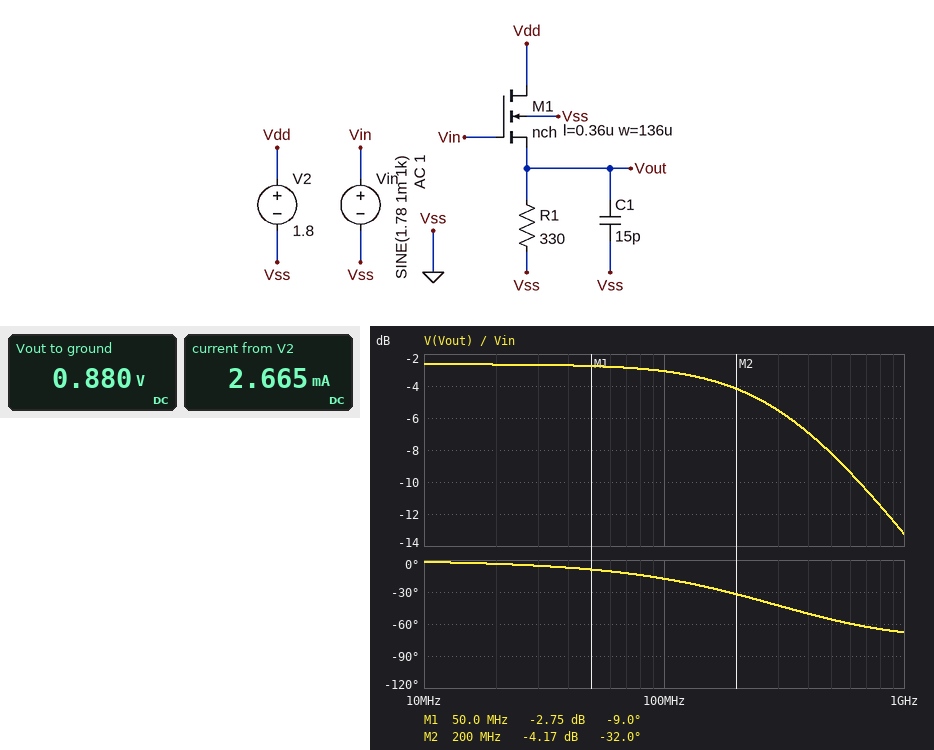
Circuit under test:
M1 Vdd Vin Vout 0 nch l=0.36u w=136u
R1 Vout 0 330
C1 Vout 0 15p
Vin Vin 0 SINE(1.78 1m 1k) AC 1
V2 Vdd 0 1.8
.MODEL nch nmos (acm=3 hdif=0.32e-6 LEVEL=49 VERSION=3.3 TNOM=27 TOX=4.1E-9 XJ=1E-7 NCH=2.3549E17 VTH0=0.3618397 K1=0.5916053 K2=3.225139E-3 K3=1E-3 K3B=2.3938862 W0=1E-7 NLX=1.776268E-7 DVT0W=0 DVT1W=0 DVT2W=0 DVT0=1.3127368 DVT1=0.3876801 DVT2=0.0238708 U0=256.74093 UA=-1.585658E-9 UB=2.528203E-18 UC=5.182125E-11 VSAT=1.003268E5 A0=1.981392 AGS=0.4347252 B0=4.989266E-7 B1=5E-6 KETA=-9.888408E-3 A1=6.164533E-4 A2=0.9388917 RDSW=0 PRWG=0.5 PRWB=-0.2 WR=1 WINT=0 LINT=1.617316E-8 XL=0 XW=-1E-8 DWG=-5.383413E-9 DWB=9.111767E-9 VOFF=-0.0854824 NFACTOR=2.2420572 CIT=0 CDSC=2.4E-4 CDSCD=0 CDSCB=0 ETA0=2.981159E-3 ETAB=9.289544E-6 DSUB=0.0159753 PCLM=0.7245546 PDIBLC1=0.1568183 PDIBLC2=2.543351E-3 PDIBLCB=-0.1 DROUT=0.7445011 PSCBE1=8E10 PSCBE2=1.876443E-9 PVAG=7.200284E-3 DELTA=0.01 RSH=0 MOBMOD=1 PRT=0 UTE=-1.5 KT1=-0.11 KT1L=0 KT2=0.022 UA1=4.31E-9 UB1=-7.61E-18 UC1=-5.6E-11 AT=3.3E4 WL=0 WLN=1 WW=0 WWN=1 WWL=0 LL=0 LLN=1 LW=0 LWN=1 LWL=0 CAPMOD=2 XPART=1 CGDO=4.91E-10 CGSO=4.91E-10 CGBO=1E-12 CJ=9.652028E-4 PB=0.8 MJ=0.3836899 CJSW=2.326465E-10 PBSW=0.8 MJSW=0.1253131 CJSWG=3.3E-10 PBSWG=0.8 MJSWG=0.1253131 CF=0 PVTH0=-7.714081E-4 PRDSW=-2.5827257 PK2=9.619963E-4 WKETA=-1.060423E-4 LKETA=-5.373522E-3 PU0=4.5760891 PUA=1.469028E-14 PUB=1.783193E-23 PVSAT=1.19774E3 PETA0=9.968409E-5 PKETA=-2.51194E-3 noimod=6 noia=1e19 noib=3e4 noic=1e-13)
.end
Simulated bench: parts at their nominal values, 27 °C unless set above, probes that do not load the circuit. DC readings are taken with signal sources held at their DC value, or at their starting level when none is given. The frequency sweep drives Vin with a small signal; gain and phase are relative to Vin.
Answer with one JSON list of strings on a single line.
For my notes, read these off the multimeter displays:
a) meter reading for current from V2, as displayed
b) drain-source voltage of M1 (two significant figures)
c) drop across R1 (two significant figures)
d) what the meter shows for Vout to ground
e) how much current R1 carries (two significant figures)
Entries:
["2.665 mA", "920 mV", "880 mV", "0.880 V", "2.7 mA"]
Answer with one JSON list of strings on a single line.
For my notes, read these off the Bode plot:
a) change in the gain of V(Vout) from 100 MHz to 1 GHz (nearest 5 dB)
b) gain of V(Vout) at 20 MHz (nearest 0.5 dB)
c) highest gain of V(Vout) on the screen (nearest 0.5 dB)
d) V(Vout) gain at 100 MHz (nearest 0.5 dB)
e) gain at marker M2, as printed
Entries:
["-10 dB", "-2.5 dB", "-2.5 dB", "-3.0 dB", "-4.17 dB"]
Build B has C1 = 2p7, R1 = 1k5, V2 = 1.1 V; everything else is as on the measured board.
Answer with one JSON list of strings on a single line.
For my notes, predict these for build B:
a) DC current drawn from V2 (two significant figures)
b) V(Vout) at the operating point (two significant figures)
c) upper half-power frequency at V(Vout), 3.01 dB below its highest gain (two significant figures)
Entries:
["650 µA", "970 mV", "670 MHz"]
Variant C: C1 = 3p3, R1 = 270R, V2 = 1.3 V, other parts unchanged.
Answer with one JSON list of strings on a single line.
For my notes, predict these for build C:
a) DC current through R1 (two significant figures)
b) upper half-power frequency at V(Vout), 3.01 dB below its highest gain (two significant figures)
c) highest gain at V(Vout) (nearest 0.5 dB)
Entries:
["3.2 mA", "1.4 GHz", "-3.0 dB"]
